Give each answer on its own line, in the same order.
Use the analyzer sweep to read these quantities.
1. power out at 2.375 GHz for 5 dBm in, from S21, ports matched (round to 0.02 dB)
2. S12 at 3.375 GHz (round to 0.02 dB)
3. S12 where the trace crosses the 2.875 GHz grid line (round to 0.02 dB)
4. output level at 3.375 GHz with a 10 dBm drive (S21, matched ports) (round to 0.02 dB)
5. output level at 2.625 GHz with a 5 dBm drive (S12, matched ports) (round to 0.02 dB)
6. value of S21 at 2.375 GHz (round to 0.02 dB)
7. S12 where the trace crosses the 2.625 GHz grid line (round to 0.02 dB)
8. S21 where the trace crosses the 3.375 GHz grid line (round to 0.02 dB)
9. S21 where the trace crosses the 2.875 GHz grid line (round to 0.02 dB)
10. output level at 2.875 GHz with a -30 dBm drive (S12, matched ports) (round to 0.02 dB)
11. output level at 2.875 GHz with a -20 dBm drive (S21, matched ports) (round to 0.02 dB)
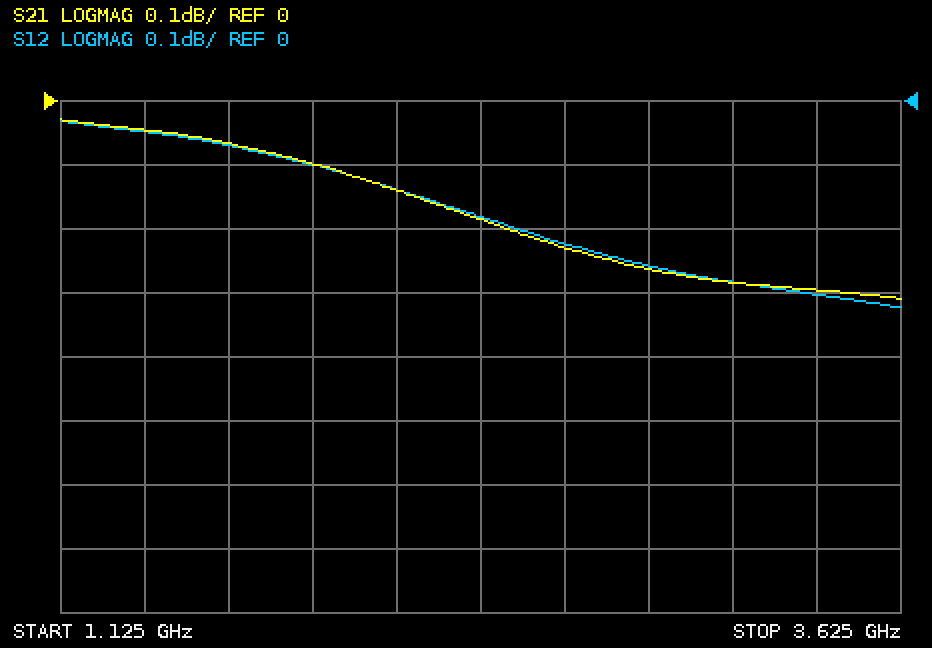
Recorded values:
4.82 dBm
-0.30 dB
-0.26 dB
9.70 dBm
4.78 dBm
-0.18 dB
-0.22 dB
-0.30 dB
-0.26 dB
-30.26 dBm
-20.26 dBm
